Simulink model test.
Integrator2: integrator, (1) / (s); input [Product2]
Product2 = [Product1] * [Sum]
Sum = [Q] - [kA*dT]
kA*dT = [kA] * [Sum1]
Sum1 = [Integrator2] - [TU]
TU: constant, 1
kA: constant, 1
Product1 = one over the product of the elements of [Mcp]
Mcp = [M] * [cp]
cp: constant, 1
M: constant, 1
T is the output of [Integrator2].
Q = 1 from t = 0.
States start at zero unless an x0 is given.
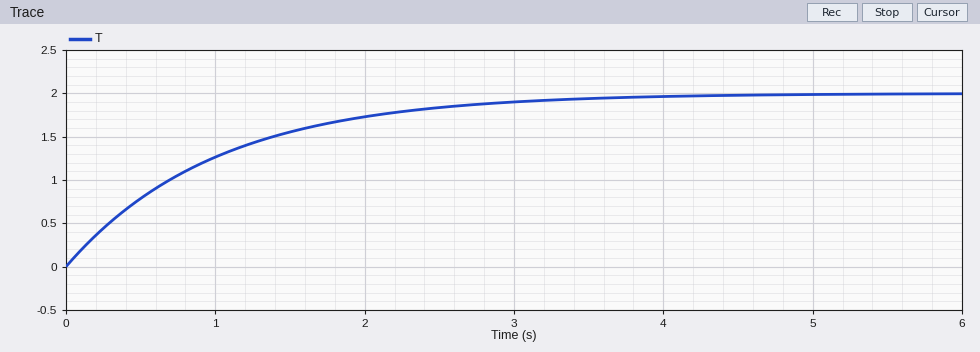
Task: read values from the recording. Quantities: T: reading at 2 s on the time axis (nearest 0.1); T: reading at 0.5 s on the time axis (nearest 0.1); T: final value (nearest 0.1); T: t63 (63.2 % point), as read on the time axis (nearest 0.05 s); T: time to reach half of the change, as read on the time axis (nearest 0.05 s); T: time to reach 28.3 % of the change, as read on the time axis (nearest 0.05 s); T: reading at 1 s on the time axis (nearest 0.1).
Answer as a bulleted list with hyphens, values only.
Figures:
- 1.7
- 0.8
- 2.0
- 1.00 s
- 0.70 s
- 0.35 s
- 1.3
